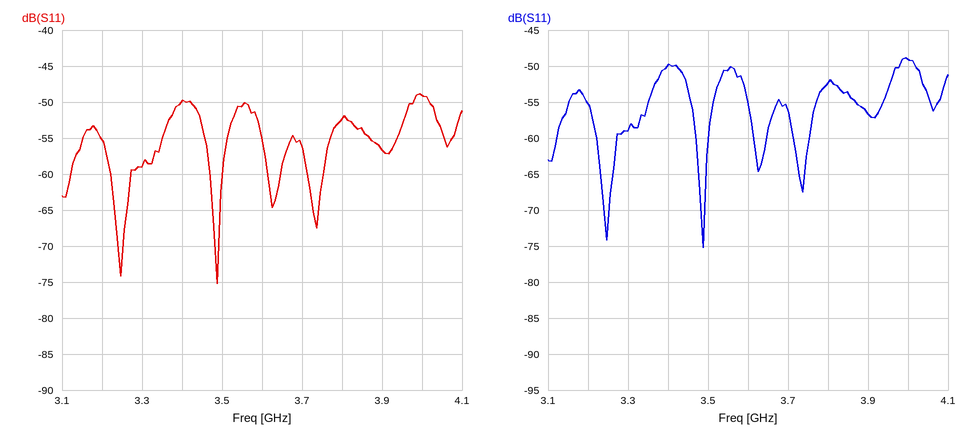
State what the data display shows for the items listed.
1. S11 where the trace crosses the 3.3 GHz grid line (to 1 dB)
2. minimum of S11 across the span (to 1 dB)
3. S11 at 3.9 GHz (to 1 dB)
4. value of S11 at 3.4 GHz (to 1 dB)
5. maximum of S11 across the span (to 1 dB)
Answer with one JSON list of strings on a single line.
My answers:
["-59 dB", "-75 dB", "-57 dB", "-50 dB", "-49 dB"]
